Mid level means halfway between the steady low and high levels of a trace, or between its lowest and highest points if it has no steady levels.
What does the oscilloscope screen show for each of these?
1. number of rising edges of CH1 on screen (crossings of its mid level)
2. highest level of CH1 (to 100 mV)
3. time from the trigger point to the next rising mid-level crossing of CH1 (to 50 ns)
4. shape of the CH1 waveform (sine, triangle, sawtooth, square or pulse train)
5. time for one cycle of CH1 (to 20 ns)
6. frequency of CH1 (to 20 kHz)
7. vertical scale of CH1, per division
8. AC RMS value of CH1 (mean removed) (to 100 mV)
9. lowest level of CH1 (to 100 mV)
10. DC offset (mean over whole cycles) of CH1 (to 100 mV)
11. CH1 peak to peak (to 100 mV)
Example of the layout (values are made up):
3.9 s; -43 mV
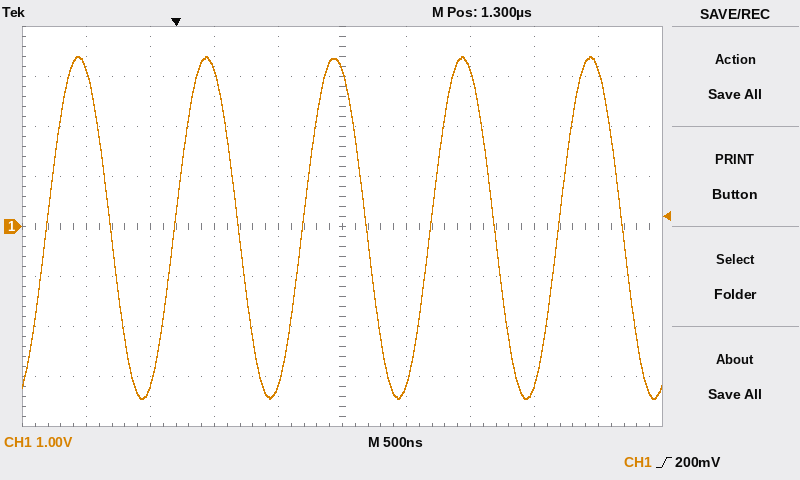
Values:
5; 3.4 V; 1.00 µs; sine; 1.00 µs; 1.00 MHz; 1 V; 2.4 V; -3.4 V; 0.0 V; 6.8 V
